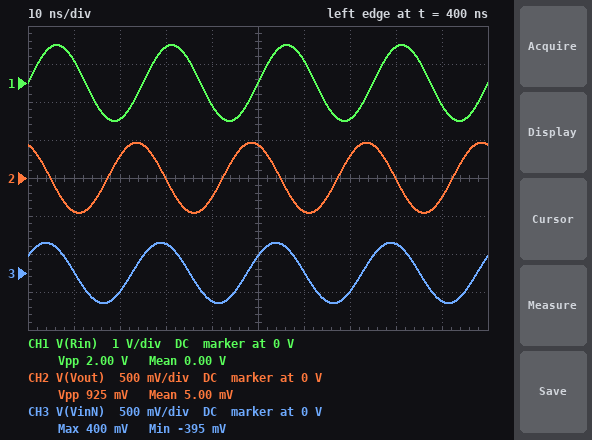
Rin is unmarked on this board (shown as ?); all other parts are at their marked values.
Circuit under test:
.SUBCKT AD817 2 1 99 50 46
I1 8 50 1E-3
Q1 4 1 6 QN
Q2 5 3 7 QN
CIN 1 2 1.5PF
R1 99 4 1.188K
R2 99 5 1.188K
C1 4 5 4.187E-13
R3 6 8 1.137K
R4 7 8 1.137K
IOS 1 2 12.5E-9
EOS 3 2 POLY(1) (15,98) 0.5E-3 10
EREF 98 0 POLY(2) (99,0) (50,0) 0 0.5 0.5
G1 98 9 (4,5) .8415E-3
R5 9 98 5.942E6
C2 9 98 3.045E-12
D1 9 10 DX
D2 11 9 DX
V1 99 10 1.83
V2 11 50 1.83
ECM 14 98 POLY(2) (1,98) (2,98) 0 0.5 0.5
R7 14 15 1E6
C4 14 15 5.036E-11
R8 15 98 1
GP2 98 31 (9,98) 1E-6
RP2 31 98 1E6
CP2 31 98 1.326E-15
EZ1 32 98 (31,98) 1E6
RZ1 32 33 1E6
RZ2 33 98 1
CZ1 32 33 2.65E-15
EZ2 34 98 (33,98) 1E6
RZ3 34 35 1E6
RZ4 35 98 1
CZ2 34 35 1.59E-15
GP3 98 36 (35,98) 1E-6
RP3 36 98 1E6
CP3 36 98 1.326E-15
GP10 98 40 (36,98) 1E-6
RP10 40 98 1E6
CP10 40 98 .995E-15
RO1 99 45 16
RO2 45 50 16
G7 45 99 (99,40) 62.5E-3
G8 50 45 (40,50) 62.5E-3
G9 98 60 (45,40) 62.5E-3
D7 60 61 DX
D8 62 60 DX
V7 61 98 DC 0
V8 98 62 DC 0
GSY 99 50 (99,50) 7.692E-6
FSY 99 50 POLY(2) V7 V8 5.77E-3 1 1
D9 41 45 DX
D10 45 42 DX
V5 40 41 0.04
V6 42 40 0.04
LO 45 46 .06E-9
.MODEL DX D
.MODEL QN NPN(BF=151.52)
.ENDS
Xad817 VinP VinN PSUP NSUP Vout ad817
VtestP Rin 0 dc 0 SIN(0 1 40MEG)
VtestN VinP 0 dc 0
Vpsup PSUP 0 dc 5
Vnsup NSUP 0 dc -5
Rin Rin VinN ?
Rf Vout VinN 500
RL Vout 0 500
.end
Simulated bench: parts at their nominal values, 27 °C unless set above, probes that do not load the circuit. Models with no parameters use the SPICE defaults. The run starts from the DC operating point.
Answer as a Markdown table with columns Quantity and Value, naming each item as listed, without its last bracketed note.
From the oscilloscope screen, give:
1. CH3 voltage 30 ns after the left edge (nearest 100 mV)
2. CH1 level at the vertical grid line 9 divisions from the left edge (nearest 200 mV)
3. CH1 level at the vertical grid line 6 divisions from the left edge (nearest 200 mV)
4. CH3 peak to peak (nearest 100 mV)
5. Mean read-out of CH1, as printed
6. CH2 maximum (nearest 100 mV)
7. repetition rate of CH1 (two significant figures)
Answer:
| Quantity | Value |
|---|---|
| CH3 voltage 30 ns after the left edge | 400 mV |
| CH1 level at the vertical grid line 9 divisions from the left edge | -600 mV |
| CH1 level at the vertical grid line 6 divisions from the left edge | 600 mV |
| CH3 peak to peak | 800 mV |
| Mean read-out of CH1, as printed | 0.00 V |
| CH2 maximum | 500 mV |
| repetition rate of CH1 | 40 MHz |
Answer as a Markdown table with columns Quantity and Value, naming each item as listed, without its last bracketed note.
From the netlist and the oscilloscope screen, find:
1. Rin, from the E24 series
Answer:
| Quantity | Value |
|---|---|
| Rin, from the E24 series | 750 Ω |
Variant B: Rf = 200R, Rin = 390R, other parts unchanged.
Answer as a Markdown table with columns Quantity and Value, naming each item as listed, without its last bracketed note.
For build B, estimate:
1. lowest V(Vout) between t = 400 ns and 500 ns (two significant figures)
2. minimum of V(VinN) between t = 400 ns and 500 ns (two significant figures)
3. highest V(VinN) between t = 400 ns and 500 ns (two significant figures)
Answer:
| Quantity | Value |
|---|---|
| lowest V(Vout) between t = 400 ns and 500 ns | -370 mV |
| minimum of V(VinN) between t = 400 ns and 500 ns | -320 mV |
| highest V(VinN) between t = 400 ns and 500 ns | 320 mV |
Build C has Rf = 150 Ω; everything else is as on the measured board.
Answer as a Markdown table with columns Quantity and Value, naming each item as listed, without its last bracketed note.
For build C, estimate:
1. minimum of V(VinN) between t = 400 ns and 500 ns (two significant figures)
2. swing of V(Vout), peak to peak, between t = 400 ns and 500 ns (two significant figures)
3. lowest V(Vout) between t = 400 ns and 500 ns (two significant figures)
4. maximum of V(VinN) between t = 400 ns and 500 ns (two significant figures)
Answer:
| Quantity | Value |
|---|---|
| minimum of V(VinN) between t = 400 ns and 500 ns | -150 mV |
| swing of V(Vout), peak to peak, between t = 400 ns and 500 ns | 330 mV |
| lowest V(Vout) between t = 400 ns and 500 ns | -160 mV |
| maximum of V(VinN) between t = 400 ns and 500 ns | 150 mV |
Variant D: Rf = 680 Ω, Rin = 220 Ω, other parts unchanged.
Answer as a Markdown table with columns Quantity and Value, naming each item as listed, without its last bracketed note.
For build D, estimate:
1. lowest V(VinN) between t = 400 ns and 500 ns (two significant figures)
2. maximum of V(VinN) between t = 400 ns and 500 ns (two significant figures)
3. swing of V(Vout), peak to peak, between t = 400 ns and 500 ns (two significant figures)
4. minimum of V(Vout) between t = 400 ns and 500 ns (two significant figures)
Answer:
| Quantity | Value |
|---|---|
| lowest V(VinN) between t = 400 ns and 500 ns | -790 mV |
| maximum of V(VinN) between t = 400 ns and 500 ns | 790 mV |
| swing of V(Vout), peak to peak, between t = 400 ns and 500 ns | 1.8 V |
| minimum of V(Vout) between t = 400 ns and 500 ns | -910 mV |
